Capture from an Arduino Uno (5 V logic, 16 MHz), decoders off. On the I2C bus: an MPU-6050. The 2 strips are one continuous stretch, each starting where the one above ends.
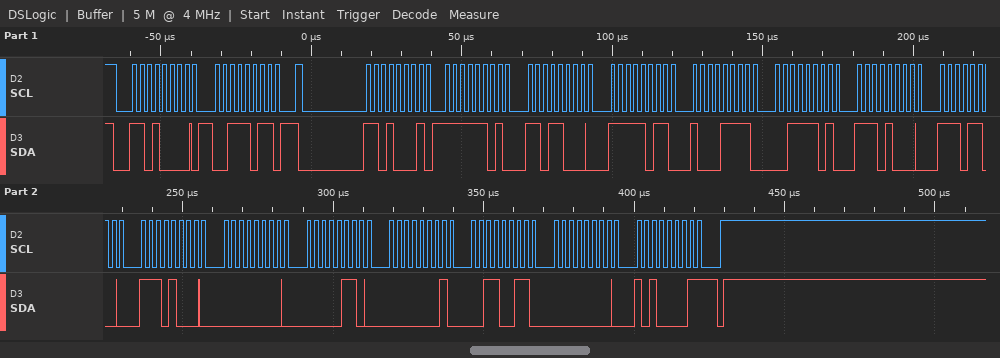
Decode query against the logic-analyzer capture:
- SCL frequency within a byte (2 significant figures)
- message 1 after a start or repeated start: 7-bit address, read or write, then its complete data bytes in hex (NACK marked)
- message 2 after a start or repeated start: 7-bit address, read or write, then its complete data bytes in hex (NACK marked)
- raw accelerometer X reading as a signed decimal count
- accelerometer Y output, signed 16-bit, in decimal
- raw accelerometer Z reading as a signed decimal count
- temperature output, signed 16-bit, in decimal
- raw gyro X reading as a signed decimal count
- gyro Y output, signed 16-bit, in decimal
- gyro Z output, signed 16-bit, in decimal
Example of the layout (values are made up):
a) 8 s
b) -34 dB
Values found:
a) 400 kHz
b) 0x68 write: 3B
c) 0x68 read: FD D8 FB 8F 3D E8 EC E8 00 06 01 33 00 A1 NACK
d) -552
e) -1137
f) 15848
g) -4888
h) 6
i) 307
j) 161
